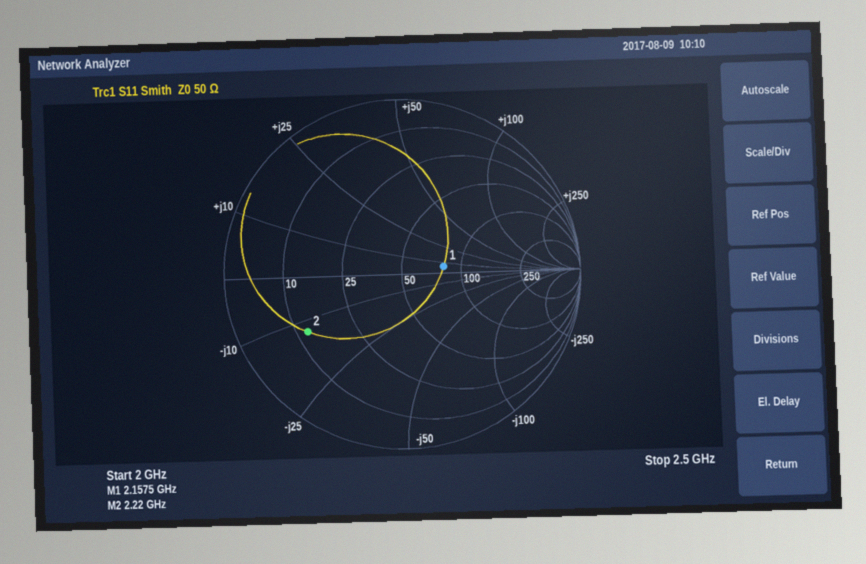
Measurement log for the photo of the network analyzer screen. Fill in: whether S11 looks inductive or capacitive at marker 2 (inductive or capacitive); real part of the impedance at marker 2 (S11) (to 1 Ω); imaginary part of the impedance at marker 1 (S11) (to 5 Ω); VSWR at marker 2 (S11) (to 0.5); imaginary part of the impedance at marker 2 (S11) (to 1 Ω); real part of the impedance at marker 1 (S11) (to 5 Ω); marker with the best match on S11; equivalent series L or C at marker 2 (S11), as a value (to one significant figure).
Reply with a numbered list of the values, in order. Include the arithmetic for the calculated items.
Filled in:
1. capacitive
2. 12 Ω
3. +5 Ω
4. 4.5
5. -13 Ω
6. 80 Ω
7. marker 1
8. C = 1/(2π × 2.22 GHz × 13 Ω) ≈ 6 pF
